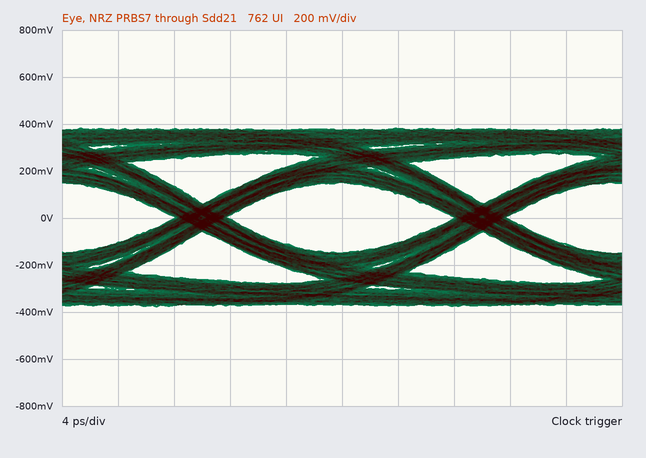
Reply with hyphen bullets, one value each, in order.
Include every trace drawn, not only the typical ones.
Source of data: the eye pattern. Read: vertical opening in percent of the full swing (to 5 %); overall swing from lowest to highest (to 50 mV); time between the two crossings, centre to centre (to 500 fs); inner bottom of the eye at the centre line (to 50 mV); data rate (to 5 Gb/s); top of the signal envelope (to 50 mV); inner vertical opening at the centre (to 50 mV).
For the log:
- 40 %
- 750 mV
- 20.0 ps
- -150 mV
- 50 Gb/s
- 400 mV
- 300 mV
